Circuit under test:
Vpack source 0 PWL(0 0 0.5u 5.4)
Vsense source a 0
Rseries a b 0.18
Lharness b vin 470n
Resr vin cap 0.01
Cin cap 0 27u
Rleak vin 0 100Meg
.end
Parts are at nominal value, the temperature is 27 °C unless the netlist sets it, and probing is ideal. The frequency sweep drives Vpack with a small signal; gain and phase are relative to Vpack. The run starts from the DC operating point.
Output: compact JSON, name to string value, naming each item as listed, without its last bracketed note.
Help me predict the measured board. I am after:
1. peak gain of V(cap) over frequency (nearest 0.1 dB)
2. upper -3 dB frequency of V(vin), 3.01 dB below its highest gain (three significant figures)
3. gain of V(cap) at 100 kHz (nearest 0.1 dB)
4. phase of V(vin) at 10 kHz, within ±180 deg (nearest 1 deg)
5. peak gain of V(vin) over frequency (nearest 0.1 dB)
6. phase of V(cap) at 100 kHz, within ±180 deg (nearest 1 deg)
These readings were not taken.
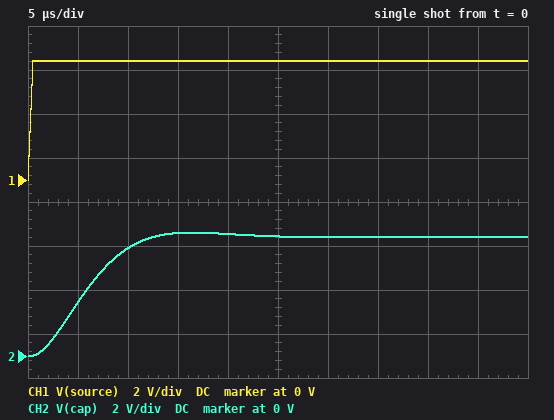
{"peak gain of V(cap) over frequency": "0 dB", "upper -3 dB frequency of V(vin), 3.01 dB below its highest gain": "44.0 kHz", "gain of V(cap) at 100 kHz": "-14.2 dB", "phase of V(vin) at 10 kHz, within ±180 deg": "-18 deg", "peak gain of V(vin) over frequency": "0 dB", "phase of V(cap) at 100 kHz, within ±180 deg": "-141 deg"}
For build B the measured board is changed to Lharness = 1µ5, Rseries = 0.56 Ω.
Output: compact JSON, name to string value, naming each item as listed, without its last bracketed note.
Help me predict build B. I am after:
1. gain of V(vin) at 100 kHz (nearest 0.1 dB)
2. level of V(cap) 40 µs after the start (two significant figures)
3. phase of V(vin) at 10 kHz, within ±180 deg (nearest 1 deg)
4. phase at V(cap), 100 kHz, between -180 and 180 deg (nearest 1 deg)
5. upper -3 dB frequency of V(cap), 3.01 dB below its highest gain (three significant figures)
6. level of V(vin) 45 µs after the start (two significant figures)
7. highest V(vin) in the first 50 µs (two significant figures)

{"gain of V(vin) at 100 kHz": "-24.9 dB", "level of V(cap) 40 µs after the start": "5.1 V", "phase of V(vin) at 10 kHz, within ±180 deg": "-48 deg", "phase at V(cap), 100 kHz, between -180 and 180 deg": "-147 deg", "upper -3 dB frequency of V(cap), 3.01 dB below its highest gain": "12.4 kHz", "level of V(vin) 45 µs after the start": "5.2 V", "highest V(vin) in the first 50 µs": "5.3 V"}
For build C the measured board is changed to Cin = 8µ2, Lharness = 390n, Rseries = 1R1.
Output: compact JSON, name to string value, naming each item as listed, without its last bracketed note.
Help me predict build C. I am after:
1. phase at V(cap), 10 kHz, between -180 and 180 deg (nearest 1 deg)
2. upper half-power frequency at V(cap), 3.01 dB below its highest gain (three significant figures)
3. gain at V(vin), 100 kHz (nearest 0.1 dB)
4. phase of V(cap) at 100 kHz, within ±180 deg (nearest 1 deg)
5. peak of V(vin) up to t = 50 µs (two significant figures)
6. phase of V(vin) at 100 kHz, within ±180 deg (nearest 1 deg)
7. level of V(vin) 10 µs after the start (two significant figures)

{"phase at V(cap), 10 kHz, between -180 and 180 deg": "-30 deg", "upper half-power frequency at V(cap), 3.01 dB below its highest gain": "18.2 kHz", "gain at V(vin), 100 kHz": "-15.1 dB", "phase of V(cap) at 100 kHz, within ±180 deg": "-93 deg", "peak of V(vin) up to t = 50 µs": "5.4 V", "phase of V(vin) at 100 kHz, within ±180 deg": "-90 deg", "level of V(vin) 10 µs after the start": "3.6 V"}
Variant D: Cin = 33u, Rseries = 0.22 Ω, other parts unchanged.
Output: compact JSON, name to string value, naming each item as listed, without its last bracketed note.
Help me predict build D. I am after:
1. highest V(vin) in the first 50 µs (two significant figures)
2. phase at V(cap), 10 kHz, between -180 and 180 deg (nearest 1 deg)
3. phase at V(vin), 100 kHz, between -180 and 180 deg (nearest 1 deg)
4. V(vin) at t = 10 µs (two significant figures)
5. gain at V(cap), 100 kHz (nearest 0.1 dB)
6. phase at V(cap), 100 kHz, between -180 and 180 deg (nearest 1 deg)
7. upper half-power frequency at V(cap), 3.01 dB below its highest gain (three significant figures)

{"highest V(vin) in the first 50 µs": "5.4 V", "phase at V(cap), 10 kHz, between -180 and 180 deg": "-27 deg", "phase at V(vin), 100 kHz, between -180 and 180 deg": "-125 deg", "V(vin) at t = 10 µs": "4.0 V", "gain at V(cap), 100 kHz": "-16.9 dB", "phase at V(cap), 100 kHz, between -180 and 180 deg": "-137 deg", "upper half-power frequency at V(cap), 3.01 dB below its highest gain": "27.4 kHz"}
